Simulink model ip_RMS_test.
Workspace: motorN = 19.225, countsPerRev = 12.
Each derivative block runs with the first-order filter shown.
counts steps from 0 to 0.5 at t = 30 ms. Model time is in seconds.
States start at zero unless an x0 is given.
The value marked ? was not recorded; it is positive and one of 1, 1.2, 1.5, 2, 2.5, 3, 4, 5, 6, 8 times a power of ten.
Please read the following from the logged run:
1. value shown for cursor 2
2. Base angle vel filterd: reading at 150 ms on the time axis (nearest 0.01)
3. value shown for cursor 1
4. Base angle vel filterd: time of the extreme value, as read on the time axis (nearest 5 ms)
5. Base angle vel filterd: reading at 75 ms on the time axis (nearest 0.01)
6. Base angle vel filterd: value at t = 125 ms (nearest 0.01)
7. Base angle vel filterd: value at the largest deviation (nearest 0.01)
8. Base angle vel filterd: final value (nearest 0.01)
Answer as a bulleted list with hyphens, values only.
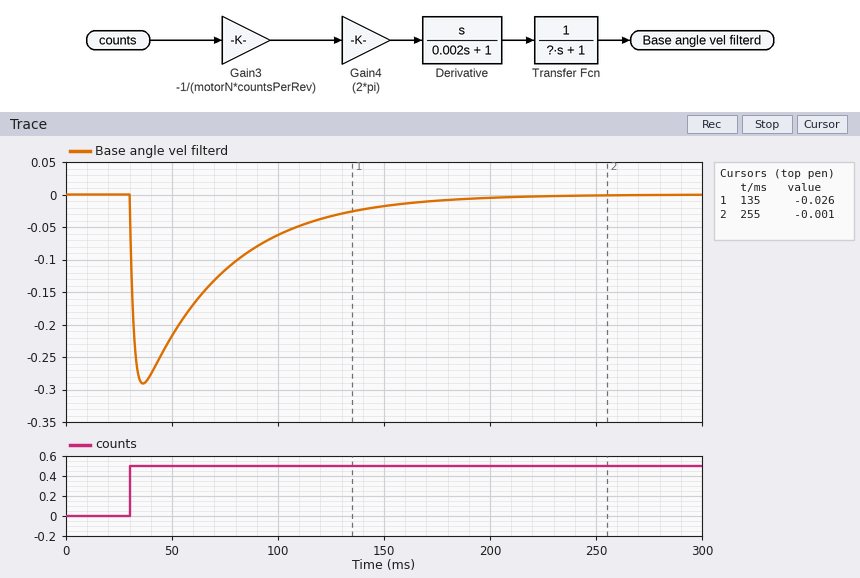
- -0.001
- -0.02
- -0.026
- 35 ms
- -0.12
- -0.03
- -0.29
- 0.00
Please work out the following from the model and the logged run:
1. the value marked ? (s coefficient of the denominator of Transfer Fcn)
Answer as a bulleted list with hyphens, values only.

- 0.04
